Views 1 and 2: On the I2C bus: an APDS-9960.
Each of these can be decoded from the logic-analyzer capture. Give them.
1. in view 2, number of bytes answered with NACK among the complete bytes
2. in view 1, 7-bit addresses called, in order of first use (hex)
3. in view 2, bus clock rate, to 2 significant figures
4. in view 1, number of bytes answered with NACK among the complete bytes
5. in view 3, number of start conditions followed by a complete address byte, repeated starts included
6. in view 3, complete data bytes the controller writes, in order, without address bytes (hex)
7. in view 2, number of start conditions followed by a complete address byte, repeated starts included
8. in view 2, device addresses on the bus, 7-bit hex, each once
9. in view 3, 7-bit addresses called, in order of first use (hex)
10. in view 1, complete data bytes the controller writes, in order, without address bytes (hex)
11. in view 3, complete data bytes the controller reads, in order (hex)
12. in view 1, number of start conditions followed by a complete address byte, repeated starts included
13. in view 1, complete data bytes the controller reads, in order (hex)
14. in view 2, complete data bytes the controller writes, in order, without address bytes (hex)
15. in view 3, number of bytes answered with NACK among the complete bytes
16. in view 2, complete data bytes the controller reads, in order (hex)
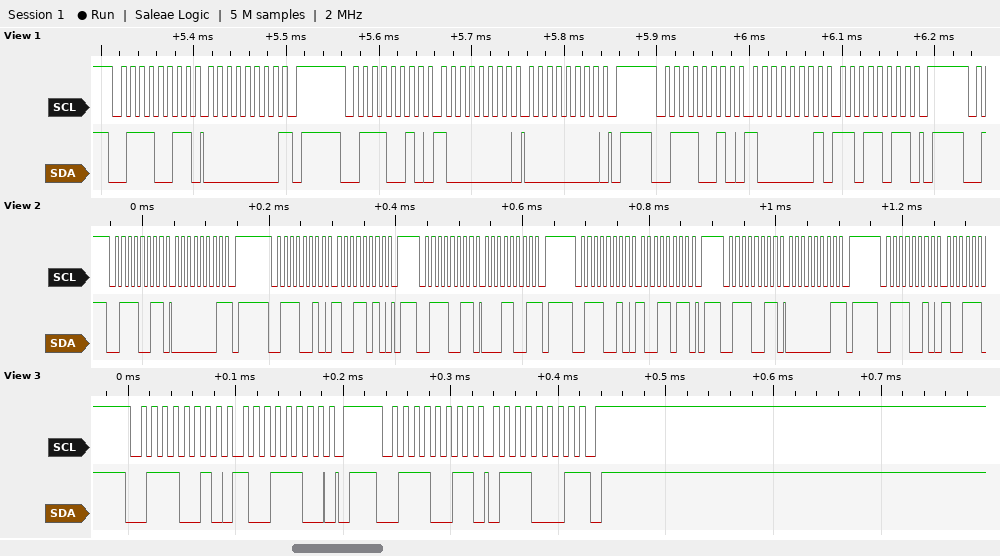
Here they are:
3
0x39
100 kHz
1
2
9C
6
0x39
0x39
80 00 81 DB
71
3
00
9A 9B
1
01 19 01
